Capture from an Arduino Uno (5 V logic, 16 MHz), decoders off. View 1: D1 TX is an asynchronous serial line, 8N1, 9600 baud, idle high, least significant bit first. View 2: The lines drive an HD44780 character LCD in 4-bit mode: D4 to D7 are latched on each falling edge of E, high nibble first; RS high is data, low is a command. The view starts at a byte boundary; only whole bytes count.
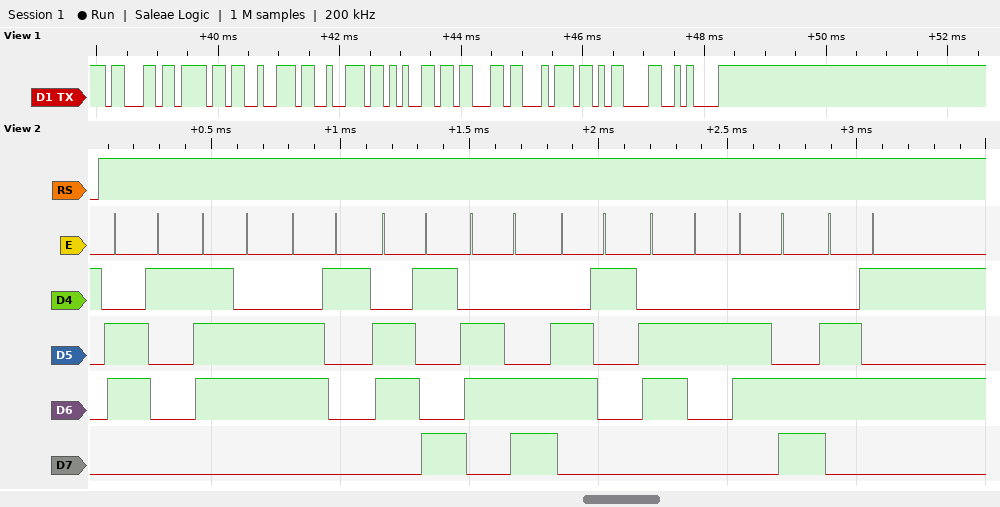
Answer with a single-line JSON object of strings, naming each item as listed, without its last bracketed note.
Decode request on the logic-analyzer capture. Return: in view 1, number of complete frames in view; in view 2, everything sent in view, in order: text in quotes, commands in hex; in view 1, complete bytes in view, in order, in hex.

{"in view 1, number of complete frames in view": "9", "in view 2, everything sent in view, in order: text in quotes, commands in hex": "\"available\"", "in view 1, complete bytes in view, in order, in hex": "63 6F 72 72 65 63 74 0D 0A"}
